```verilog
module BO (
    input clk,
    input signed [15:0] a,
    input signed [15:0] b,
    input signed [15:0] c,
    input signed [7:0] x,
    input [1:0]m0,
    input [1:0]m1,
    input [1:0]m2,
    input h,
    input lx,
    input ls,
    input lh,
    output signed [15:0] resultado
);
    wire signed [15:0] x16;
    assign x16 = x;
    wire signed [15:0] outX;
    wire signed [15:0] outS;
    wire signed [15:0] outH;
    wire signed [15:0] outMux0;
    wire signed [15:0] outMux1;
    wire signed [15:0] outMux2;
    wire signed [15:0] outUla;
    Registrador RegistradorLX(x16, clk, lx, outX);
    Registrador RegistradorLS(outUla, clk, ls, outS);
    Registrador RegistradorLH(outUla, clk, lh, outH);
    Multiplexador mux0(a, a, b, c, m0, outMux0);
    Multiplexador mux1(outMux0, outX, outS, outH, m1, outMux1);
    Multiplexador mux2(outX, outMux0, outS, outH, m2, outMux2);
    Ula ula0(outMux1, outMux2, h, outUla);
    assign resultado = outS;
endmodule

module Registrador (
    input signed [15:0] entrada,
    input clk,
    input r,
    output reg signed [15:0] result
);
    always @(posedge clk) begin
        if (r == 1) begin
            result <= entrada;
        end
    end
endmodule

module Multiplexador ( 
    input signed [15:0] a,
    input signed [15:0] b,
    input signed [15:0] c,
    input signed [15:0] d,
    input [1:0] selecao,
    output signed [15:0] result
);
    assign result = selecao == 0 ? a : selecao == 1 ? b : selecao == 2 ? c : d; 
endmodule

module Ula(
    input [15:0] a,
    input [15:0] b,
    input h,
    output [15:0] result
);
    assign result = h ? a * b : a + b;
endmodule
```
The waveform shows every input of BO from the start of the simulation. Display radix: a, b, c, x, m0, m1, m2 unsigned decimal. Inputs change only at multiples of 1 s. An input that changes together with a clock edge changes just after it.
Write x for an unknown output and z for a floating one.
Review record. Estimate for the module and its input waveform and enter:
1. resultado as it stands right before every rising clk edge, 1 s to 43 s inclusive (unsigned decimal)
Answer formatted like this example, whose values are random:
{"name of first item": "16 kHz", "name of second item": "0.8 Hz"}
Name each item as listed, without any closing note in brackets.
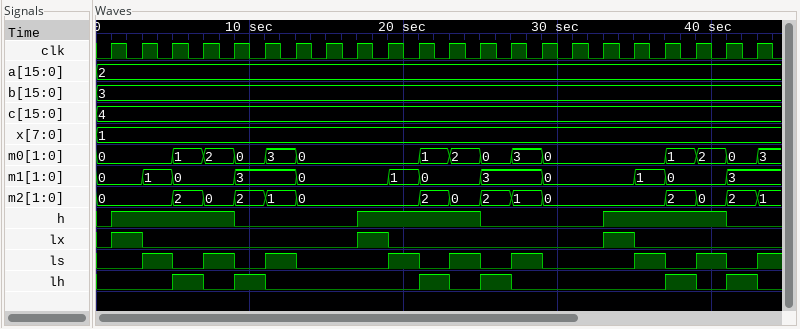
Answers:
{"resultado as it stands right before every rising clk edge, 1 s to 43 s inclusive": "x, x, x, 1, 1, 3, 3, 9, 9, 9, 9, 1, 1, 3, 3, 9, 9, 9, 9, 1, 1, 3"}
